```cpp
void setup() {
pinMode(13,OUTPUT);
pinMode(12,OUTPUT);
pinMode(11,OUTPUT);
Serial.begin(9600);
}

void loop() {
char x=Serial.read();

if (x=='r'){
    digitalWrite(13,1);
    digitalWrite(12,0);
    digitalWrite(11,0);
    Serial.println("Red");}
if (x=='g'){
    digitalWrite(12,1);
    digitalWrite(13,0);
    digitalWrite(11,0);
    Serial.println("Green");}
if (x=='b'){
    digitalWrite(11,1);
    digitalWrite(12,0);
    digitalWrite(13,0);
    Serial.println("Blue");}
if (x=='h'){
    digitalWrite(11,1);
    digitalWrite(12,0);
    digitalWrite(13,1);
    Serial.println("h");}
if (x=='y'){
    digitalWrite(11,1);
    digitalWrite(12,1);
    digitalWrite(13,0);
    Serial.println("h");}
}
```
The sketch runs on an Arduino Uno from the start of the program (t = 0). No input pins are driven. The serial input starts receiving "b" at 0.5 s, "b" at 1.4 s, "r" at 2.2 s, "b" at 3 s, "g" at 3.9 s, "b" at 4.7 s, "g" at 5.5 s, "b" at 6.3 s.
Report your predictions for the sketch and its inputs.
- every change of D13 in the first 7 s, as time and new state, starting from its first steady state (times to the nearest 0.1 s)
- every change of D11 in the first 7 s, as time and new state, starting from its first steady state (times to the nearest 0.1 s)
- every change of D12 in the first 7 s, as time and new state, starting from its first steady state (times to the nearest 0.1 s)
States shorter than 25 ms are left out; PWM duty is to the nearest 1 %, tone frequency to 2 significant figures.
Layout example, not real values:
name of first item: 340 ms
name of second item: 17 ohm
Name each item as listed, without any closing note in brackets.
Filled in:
every change of D13 in the first 7 s, as time and new state, starting from its first steady state: 0 s low; 2.2 s high; 3 s low
every change of D11 in the first 7 s, as time and new state, starting from its first steady state: 0 s low; 0.5 s high; 2.2 s low; 3 s high; 3.9 s low; 4.7 s high; 5.5 s low; 6.3 s high
every change of D12 in the first 7 s, as time and new state, starting from its first steady state: 0 s low; 3.9 s high; 4.7 s low; 5.5 s high; 6.3 s low
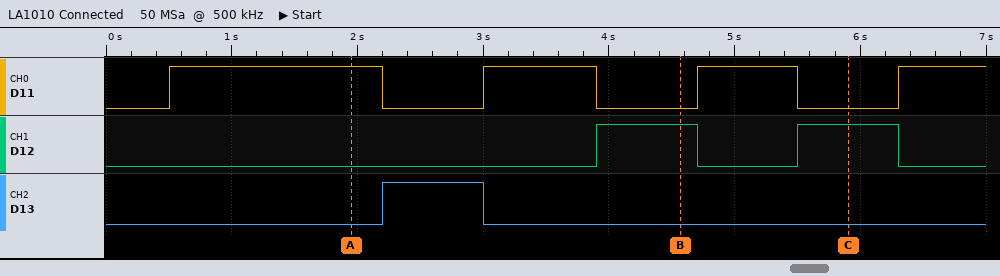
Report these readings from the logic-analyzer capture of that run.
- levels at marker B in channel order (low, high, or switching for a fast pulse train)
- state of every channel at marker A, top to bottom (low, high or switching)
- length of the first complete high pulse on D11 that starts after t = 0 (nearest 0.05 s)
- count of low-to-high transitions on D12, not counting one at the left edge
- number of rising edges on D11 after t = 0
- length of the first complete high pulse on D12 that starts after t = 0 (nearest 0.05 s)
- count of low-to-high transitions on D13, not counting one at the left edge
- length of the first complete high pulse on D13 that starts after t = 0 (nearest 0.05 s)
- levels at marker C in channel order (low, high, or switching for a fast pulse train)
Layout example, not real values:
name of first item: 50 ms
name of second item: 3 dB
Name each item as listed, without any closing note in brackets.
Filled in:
levels at marker B in channel order: D11 low, D12 high, D13 low
state of every channel at marker A, top to bottom: D11 high, D12 low, D13 low
length of the first complete high pulse on D11 that starts after t = 0: 1.70 s
count of low-to-high transitions on D12, not counting one at the left edge: 2
number of rising edges on D11 after t = 0: 4
length of the first complete high pulse on D12 that starts after t = 0: 0.80 s
count of low-to-high transitions on D13, not counting one at the left edge: 1
length of the first complete high pulse on D13 that starts after t = 0: 0.80 s
levels at marker C in channel order: D11 low, D12 high, D13 low
